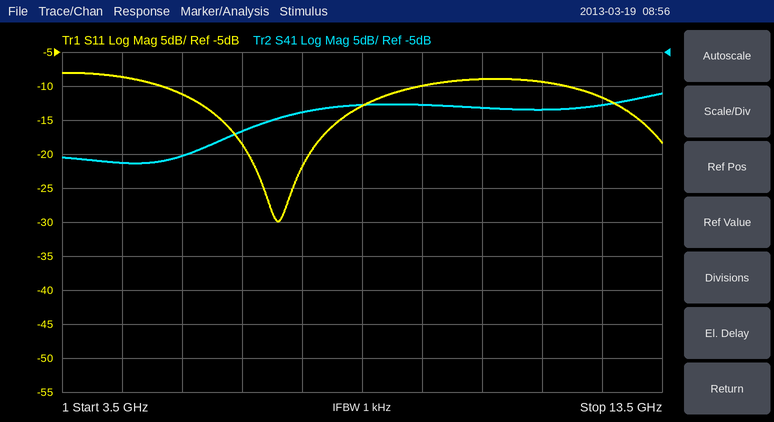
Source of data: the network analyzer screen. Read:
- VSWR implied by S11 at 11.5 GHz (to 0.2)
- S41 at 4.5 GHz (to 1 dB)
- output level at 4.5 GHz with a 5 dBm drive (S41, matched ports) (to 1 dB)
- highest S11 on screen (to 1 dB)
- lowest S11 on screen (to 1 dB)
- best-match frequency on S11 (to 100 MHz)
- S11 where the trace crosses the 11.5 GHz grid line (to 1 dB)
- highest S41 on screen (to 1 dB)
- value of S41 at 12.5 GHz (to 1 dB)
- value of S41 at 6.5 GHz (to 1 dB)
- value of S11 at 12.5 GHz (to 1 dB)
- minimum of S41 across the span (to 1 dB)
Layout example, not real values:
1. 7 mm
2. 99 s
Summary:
1. 2.0
2. -21 dB
3. -16 dBm
4. -8 dB
5. -30 dB
6. 7.1 GHz
7. -9 dB
8. -11 dB
9. -13 dB
10. -17 dB
11. -12 dB
12. -21 dB
